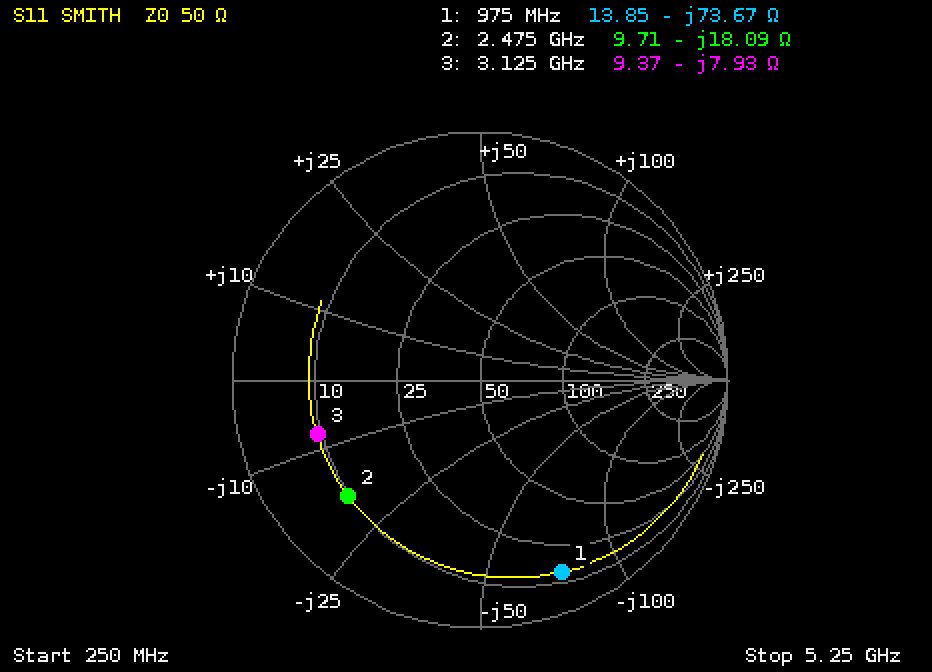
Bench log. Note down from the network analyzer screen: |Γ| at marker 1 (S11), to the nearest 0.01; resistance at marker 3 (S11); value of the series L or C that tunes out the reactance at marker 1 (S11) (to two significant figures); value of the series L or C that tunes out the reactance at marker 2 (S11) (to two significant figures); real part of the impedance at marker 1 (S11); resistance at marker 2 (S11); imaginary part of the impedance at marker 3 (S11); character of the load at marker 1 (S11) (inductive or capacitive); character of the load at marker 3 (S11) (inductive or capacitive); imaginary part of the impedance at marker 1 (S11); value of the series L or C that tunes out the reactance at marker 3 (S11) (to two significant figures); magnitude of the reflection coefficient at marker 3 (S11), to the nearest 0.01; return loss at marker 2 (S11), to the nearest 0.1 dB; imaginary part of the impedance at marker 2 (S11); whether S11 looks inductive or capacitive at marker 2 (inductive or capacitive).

0.84
9.37 Ω
12 nH
1.2 nH
13.85 Ω
9.71 Ω
-7.93 Ω
capacitive
capacitive
-73.67 Ω
400 pH
0.69
3.0 dB
-18.09 Ω
capacitive
